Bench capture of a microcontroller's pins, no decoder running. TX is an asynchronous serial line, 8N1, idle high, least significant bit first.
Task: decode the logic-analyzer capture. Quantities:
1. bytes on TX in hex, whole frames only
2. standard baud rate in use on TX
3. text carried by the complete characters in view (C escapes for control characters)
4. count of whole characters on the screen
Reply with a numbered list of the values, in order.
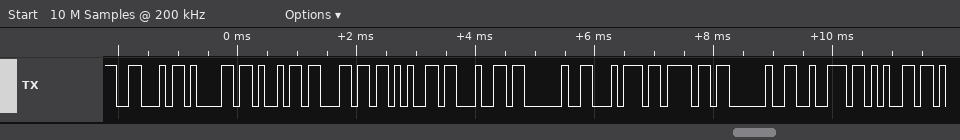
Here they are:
1. 0x46 0x61 0x69 0x6C 0x65 0x64 0x20 0x74 0x6F 0x20 0x72 0x65
2. 9600 baud
3. "Failed to re"
4. 12
